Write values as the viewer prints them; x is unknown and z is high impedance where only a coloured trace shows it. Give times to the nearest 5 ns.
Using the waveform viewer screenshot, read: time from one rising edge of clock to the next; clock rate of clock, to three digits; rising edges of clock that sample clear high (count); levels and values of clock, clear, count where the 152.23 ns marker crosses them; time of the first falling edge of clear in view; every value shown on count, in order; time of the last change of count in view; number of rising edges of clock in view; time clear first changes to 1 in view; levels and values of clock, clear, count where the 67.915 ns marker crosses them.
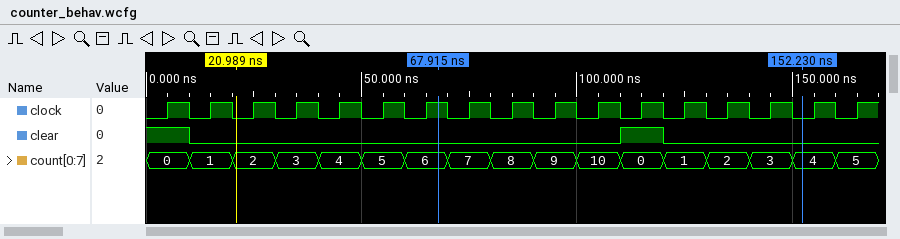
10 ns
100 MHz
2
clock=0, clear=0, count=4
10 ns
0, 1, 2, 3, 4, 5, 6, 7, 8, 9, 10, 0, 1, 2, 3, 4, 5
160 ns
17
110 ns
clock=1, clear=0, count=6
